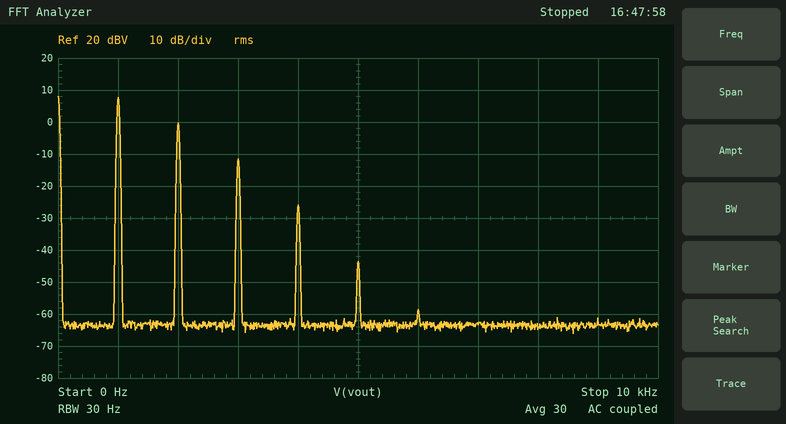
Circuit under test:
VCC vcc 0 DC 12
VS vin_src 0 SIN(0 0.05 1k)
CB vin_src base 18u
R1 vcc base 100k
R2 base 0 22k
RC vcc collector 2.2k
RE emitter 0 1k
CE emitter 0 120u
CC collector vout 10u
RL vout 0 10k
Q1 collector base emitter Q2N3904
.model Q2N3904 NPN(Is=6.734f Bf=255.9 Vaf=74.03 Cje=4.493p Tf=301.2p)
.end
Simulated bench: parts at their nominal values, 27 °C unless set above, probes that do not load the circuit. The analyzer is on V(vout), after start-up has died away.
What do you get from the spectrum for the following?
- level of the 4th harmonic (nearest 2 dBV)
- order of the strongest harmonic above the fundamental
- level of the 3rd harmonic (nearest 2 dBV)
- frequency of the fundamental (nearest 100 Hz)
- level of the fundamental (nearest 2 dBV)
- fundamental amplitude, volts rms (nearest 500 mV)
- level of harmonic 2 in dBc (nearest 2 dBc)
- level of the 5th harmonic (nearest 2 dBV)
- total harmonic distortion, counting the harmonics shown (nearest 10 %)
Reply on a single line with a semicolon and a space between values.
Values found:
-26 dBV; 2; -12 dBV; 1.0 kHz; 8 dBV; 2.5 V; -8 dBc; -44 dBV; 40 %
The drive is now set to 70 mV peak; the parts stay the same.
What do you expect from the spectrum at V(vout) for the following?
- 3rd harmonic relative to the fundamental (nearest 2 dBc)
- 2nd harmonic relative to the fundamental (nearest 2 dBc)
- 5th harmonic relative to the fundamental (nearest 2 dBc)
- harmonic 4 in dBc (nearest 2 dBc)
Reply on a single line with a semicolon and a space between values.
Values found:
-14 dBc; -6 dBc; -40 dBc; -26 dBc
